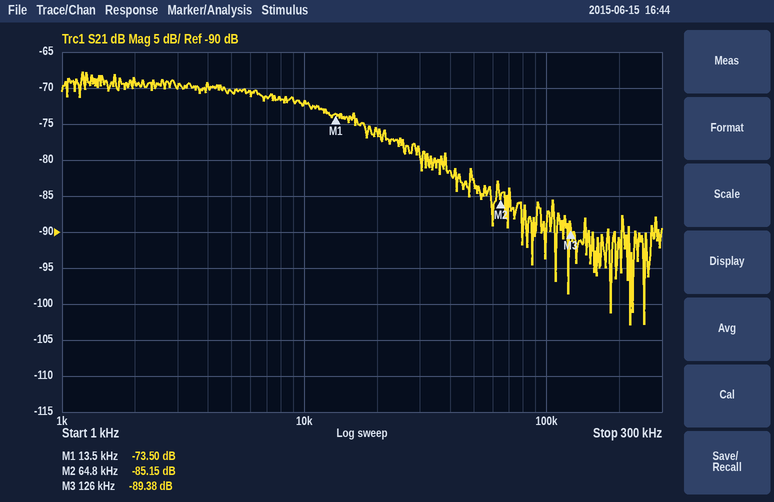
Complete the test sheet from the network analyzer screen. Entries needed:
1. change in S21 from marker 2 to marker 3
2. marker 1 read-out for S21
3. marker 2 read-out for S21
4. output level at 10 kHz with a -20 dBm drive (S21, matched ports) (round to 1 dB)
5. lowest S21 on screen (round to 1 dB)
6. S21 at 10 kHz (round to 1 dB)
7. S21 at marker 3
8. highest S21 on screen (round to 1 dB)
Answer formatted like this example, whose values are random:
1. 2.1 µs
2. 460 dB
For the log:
1. -4.23 dB
2. -73.50 dB
3. -85.15 dB
4. -92 dBm
5. -103 dB
6. -72 dB
7. -89.38 dB
8. -68 dB
